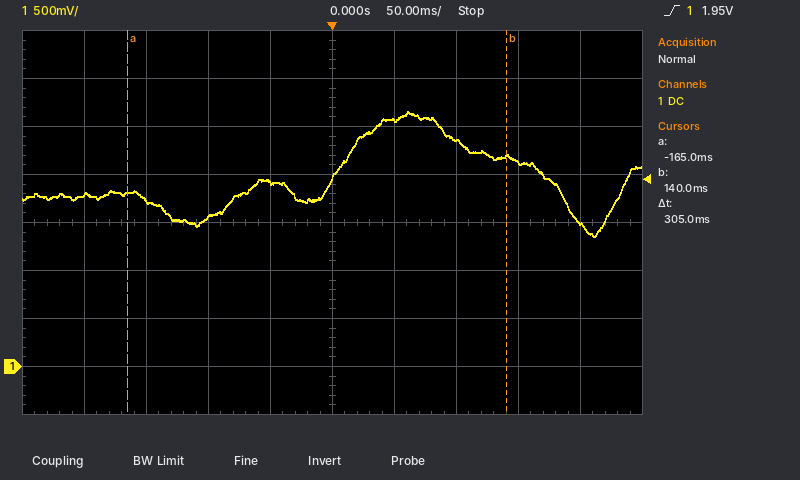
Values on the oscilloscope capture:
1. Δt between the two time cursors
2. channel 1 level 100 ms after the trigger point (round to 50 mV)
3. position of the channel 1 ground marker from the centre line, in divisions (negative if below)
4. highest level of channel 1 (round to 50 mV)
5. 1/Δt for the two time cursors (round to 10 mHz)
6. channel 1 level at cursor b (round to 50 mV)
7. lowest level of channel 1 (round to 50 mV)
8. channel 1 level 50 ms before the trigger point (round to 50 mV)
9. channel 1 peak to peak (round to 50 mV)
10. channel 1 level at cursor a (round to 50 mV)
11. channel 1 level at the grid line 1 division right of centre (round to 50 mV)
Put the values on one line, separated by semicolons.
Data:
305 ms; 2.35 V; -3.0 div; 2.65 V; 3.28 Hz; 2.20 V; 1.35 V; 1.90 V; 1.30 V; 1.80 V; 2.55 V
